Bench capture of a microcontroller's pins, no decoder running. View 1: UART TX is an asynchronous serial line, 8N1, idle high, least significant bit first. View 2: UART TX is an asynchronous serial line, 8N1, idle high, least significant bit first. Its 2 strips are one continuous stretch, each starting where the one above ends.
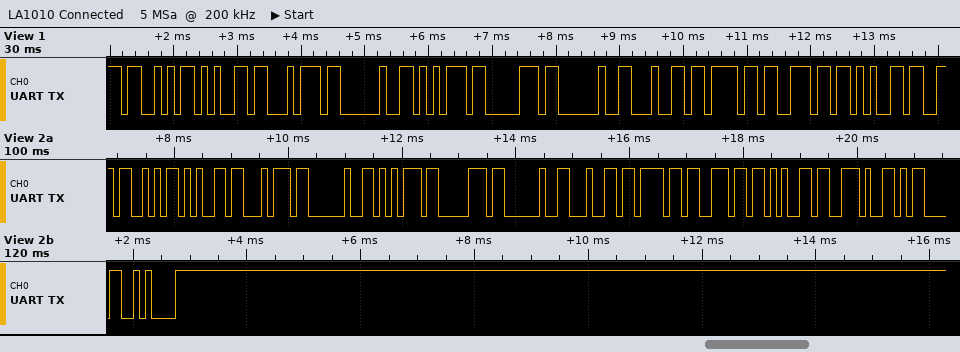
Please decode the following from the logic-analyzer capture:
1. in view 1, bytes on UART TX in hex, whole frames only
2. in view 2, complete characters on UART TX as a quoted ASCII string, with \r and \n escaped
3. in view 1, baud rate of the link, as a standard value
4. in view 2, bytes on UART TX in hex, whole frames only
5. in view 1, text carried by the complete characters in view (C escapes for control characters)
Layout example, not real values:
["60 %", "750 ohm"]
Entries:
["53 65 74 20 75 70 20 64 6F 6E 65", "\"Set up done.\\r\\n\"", "9600 baud", "0x53 0x65 0x74 0x20 0x75 0x70 0x20 0x64 0x6F 0x6E 0x65 0x2E 0x0D 0x0A", "\"Set up done\""]
